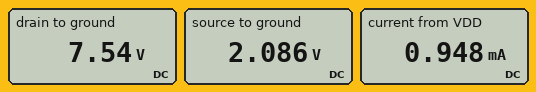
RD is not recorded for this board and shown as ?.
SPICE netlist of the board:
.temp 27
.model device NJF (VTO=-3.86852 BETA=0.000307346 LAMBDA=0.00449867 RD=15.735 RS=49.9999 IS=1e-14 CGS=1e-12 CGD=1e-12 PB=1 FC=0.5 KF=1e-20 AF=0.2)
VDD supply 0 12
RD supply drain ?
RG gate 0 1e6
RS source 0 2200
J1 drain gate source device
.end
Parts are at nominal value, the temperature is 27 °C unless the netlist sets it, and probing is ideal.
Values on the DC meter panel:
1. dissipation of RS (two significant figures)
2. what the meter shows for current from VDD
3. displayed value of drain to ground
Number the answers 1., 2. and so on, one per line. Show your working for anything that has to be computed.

1. (2.086 V)^2 / 2.2 kΩ = 2.0 mW
2. 0.948 mA
3. 7.54 V
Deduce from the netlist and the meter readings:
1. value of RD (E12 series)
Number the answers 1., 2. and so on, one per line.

1. 4.7 kΩ
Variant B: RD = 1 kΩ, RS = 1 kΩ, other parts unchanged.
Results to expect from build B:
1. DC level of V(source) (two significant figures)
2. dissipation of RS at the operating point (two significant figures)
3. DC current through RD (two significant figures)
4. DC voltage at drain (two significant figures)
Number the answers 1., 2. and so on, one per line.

1. 1.6 V
2. 2.5 mW
3. 1.6 mA
4. 10 V
